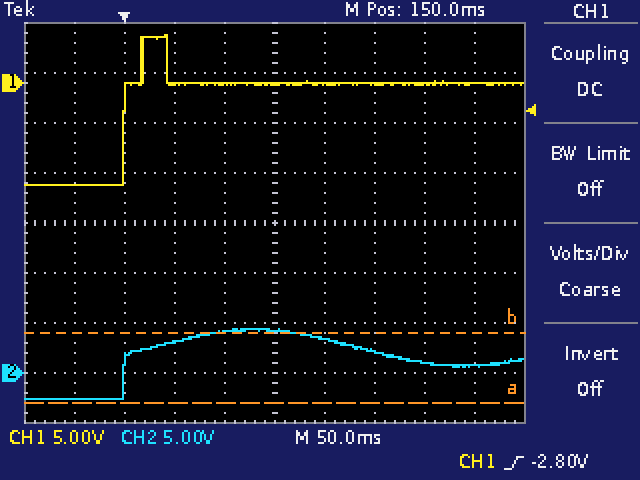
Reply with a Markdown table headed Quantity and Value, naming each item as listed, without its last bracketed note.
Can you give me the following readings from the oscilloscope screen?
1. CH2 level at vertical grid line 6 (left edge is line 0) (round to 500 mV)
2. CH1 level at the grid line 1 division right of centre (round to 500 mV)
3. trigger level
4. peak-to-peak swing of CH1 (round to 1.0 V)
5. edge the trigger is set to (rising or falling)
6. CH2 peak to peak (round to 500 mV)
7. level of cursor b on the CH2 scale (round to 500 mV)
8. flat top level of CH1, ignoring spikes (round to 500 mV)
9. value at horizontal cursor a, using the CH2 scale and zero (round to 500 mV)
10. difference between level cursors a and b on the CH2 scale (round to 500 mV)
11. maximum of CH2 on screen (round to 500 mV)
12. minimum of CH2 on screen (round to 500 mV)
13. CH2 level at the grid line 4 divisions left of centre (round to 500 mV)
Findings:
| Quantity | Value |
|---|---|
| CH2 level at vertical grid line 6 (left edge is line 0) | 3.5 V |
| CH1 level at the grid line 1 division right of centre | 0.0 V |
| trigger level | -2.80 V |
| peak-to-peak swing of CH1 | 15.0 V |
| edge the trigger is set to | rising |
| CH2 peak to peak | 7.0 V |
| level of cursor b on the CH2 scale | 4.0 V |
| flat top level of CH1, ignoring spikes | 0.0 V |
| value at horizontal cursor a, using the CH2 scale and zero | -3.0 V |
| difference between level cursors a and b on the CH2 scale | 7.0 V |
| maximum of CH2 on screen | 4.5 V |
| minimum of CH2 on screen | -2.5 V |
| CH2 level at the grid line 4 divisions left of centre | -2.5 V |
